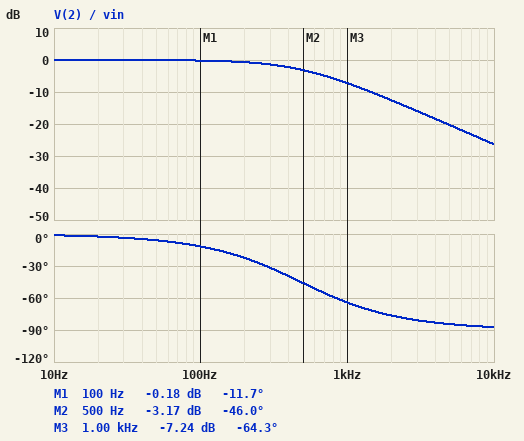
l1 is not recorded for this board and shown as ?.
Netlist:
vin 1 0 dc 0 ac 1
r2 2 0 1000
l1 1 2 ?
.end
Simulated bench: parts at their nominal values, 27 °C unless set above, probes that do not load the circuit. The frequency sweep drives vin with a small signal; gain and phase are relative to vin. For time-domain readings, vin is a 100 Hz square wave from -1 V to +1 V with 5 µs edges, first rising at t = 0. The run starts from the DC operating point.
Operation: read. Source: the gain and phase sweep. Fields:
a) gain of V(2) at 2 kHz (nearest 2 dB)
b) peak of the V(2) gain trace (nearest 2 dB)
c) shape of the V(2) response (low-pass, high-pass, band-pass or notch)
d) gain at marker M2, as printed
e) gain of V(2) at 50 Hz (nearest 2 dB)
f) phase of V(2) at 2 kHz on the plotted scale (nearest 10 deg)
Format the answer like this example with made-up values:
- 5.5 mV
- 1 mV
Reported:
- -12 dB
- 0 dB
- low-pass
- -3.17 dB
- 0 dB
- -80 deg
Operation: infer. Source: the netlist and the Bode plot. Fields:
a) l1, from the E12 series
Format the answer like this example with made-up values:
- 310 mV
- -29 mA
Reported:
- 330 mH
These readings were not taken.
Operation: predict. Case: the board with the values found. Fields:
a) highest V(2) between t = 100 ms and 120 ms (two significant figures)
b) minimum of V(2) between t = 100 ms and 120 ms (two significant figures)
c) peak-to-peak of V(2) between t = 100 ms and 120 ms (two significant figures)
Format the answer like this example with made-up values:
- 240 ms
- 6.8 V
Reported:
- 1.0 V
- -1.0 V
- 2.0 V
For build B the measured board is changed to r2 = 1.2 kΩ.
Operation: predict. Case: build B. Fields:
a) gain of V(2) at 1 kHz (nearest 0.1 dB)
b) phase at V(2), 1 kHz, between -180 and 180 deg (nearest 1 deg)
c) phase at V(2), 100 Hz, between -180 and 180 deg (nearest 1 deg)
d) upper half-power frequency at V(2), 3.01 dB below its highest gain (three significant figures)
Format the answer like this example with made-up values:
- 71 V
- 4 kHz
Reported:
- -6.0 dB
- -60 deg
- -10 deg
- 579 Hz
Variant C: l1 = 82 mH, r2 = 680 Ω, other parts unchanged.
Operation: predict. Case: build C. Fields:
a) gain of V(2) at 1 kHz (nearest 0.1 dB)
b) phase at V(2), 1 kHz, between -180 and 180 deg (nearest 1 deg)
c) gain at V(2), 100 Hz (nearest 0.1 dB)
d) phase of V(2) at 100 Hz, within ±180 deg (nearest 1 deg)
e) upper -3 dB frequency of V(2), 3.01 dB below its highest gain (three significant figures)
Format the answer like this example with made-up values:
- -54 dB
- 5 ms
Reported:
- -2.0 dB
- -37 deg
- 0 dB
- -4 deg
- 1.32 kHz
